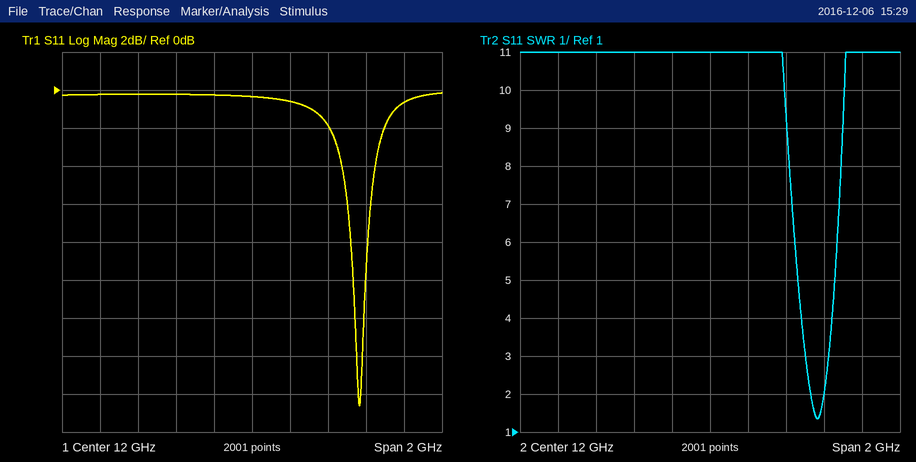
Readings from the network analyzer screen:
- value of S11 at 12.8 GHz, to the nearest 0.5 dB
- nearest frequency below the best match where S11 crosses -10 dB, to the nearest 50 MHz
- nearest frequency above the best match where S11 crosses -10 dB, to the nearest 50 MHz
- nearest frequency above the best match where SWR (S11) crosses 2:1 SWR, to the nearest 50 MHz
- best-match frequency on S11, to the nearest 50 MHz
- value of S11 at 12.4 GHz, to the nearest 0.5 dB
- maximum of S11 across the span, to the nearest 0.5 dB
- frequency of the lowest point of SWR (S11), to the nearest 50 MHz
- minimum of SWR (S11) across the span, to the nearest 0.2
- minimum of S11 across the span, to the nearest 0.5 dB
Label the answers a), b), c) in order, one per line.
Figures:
a) -0.5 dB
b) 12.55 GHz
c) 12.60 GHz
d) 12.60 GHz
e) 12.55 GHz
f) -2.0 dB
g) 0.0 dB
h) 12.55 GHz
i) 1.4
j) -16.5 dB
